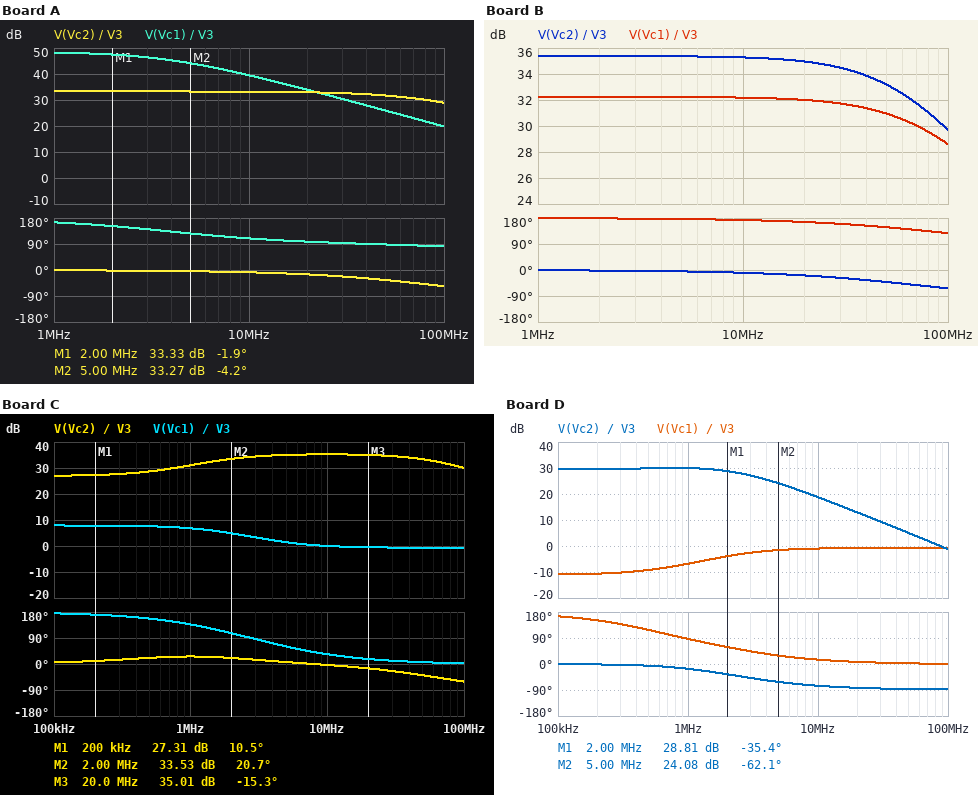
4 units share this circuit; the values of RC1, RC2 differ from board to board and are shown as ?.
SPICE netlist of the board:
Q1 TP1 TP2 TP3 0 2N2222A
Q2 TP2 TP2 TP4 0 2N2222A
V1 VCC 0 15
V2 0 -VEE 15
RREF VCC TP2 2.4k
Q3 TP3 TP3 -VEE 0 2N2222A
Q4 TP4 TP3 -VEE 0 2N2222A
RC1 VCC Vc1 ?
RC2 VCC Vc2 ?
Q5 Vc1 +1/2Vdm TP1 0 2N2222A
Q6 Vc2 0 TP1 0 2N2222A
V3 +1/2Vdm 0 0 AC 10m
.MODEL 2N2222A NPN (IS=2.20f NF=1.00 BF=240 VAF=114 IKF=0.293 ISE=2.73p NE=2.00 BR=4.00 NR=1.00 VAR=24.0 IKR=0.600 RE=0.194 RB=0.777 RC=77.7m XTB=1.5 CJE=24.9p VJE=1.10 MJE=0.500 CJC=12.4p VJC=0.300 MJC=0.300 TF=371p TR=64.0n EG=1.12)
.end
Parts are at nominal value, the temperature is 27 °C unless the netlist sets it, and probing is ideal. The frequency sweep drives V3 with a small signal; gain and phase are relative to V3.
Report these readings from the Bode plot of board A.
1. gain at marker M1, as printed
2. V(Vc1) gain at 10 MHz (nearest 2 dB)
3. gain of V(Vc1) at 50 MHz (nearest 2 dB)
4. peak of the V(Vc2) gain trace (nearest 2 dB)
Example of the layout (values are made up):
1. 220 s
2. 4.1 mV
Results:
1. 33.33 dB
2. 40 dB
3. 26 dB
4. 34 dB
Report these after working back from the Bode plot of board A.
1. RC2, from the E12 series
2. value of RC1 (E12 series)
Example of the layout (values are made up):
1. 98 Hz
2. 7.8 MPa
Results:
1. 470 Ω
2. 2.7 kΩ
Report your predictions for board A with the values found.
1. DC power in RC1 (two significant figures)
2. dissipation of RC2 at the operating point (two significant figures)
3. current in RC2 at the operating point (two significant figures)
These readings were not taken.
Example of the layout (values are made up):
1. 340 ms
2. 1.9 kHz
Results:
1. 85 mW
2. 18 mW
3. 6.2 mA
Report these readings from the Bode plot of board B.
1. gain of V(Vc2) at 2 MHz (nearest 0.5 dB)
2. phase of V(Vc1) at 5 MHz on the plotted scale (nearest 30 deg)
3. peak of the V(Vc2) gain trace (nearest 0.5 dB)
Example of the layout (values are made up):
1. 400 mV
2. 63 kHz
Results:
1. 35.5 dB
2. 180 deg
3. 35.5 dB
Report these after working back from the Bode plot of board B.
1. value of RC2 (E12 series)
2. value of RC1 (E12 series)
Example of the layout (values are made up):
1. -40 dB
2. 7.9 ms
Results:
1. 560 Ω
2. 390 Ω
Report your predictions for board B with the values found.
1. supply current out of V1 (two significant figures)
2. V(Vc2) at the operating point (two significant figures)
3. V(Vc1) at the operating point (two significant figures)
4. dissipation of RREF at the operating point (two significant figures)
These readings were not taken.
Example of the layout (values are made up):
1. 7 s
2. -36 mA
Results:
1. 24 mA
2. 12 V
3. 13 V
4. 340 mW
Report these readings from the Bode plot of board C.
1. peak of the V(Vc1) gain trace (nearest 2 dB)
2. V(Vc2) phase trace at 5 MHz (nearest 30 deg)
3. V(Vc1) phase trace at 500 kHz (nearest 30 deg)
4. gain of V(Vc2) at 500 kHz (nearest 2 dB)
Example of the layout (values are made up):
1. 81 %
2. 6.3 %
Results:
1. 8 dB
2. 0 deg
3. 150 deg
4. 28 dB
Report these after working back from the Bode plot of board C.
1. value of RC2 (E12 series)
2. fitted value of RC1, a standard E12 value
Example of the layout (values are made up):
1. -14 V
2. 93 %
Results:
1. 560 Ω
2. 3.3 kΩ
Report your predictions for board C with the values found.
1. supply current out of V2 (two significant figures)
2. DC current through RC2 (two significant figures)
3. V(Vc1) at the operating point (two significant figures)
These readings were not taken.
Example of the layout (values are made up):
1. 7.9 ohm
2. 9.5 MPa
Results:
1. 24 mA
2. 6.8 mA
3. -700 mV
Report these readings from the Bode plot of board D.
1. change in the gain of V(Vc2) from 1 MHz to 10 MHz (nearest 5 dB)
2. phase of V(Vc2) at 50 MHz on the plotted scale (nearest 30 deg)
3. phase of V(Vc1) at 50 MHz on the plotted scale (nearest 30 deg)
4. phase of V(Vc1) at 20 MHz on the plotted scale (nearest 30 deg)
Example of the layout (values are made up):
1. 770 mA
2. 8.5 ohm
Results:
1. -10 dB
2. -90 deg
3. 0 deg
4. 0 deg
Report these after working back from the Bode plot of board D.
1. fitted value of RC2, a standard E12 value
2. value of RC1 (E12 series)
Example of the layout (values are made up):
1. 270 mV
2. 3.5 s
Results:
1. 2.2 kΩ
2. 3.9 kΩ
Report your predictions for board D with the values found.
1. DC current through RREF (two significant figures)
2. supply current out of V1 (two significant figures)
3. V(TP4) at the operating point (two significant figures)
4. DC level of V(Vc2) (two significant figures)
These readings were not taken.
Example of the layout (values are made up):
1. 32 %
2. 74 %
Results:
1. 12 mA
2. 23 mA
3. -14 V
4. -620 mV
